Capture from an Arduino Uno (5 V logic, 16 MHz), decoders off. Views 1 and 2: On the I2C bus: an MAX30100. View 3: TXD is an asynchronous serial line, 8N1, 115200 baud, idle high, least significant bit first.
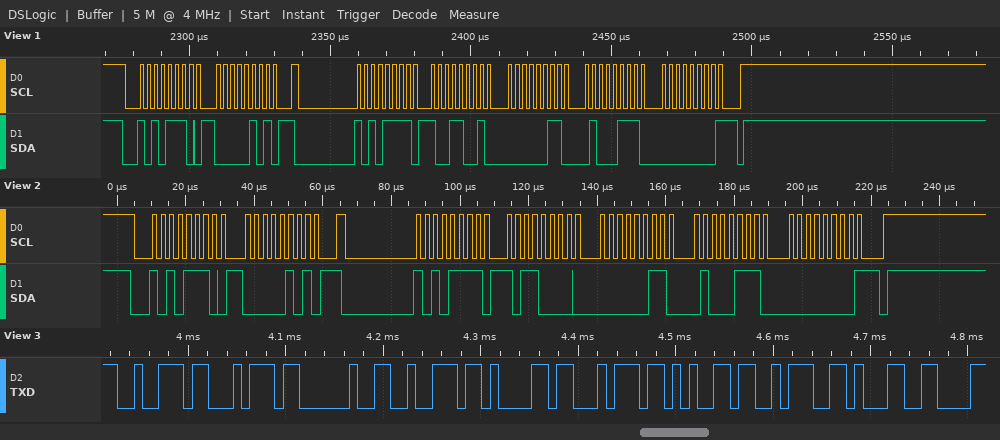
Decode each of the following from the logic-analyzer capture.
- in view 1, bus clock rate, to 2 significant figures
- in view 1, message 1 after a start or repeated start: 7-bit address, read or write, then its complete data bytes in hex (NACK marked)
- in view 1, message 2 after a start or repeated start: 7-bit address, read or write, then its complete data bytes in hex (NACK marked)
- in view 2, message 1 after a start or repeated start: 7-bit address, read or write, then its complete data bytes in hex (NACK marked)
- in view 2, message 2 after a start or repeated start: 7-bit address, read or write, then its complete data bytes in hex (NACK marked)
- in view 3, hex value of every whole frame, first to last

400 kHz
0x57 write: 05
0x57 read: 99 03 47 00 NACK
0x57 write: 05
0x57 read: B0 03 47 00 NACK
72 74 20 72 61 74 65 3A 31
